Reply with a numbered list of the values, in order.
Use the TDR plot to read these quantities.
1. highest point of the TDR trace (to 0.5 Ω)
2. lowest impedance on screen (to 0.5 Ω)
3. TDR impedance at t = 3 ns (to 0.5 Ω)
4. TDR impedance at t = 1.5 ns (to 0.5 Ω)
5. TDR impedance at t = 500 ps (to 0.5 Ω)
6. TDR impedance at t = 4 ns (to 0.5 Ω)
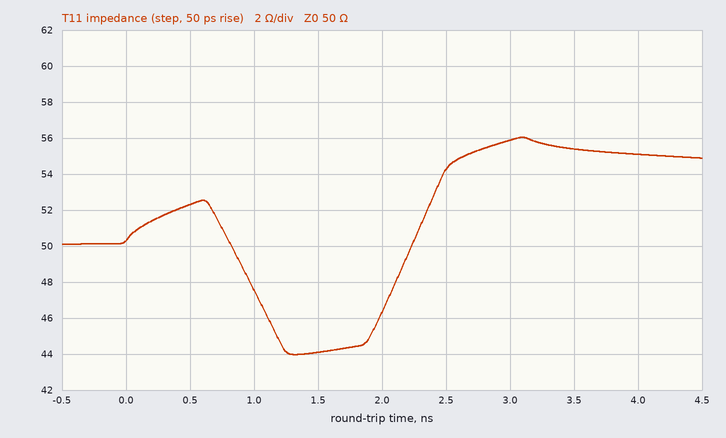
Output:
1. 56.0 Ω
2. 44.0 Ω
3. 56.0 Ω
4. 44.0 Ω
5. 52.5 Ω
6. 55.0 Ω
